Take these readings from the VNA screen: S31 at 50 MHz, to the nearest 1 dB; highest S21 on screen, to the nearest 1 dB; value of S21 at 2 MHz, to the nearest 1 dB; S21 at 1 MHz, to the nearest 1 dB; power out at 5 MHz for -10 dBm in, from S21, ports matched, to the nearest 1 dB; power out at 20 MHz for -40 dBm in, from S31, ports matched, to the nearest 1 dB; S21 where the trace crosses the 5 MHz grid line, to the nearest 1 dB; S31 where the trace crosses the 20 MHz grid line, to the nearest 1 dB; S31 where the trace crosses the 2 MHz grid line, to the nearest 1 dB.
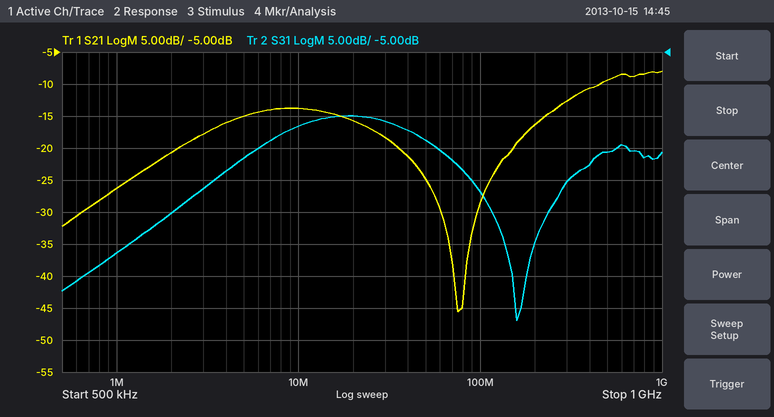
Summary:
-19 dB
-8 dB
-21 dB
-26 dB
-25 dBm
-55 dBm
-15 dB
-15 dB
-30 dB
